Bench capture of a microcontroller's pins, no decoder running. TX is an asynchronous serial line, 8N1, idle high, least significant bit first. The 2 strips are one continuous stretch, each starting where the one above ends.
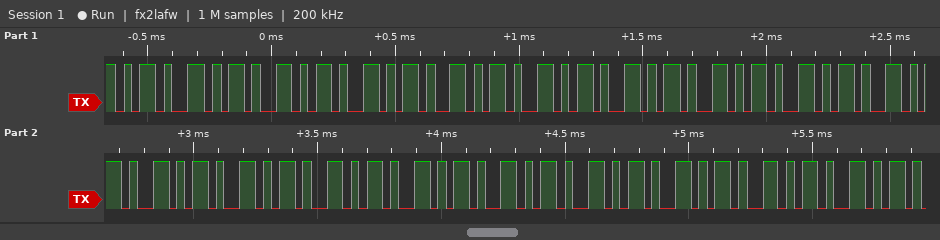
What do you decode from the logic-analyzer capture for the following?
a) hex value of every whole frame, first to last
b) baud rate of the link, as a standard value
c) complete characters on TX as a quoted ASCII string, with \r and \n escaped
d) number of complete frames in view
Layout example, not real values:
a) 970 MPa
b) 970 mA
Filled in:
a) 0x2D 0x2D 0x2D 0x2D 0x2D 0x2D 0x2D 0x2D 0x2D 0x2D 0x2D 0x2D 0x2D 0x2D 0x2D 0x2D 0x2D 0x2D
b) 31250 baud
c) "------------------"
d) 18
